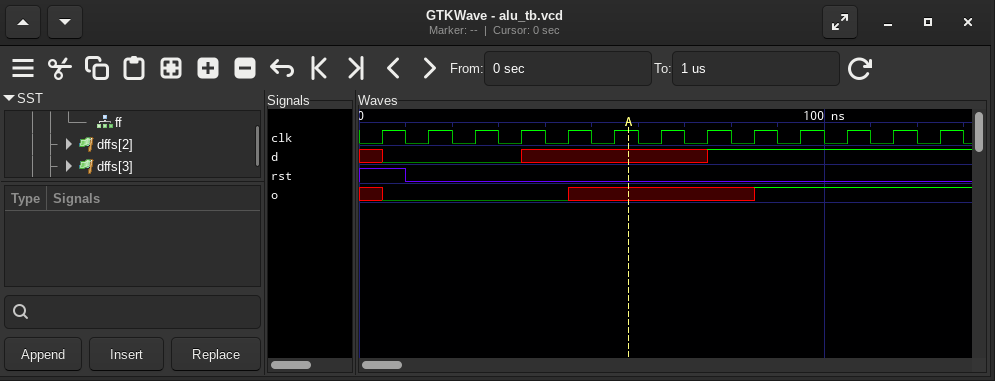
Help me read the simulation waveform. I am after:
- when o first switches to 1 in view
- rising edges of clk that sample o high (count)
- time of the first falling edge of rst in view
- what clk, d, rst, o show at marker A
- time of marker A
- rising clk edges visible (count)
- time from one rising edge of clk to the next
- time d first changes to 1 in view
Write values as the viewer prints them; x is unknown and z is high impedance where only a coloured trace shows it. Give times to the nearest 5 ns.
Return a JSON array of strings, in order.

["85 ns", "4", "10 ns", "clk=1, d=x, rst=0, o=x", "60 ns", "13", "10 ns", "75 ns"]
